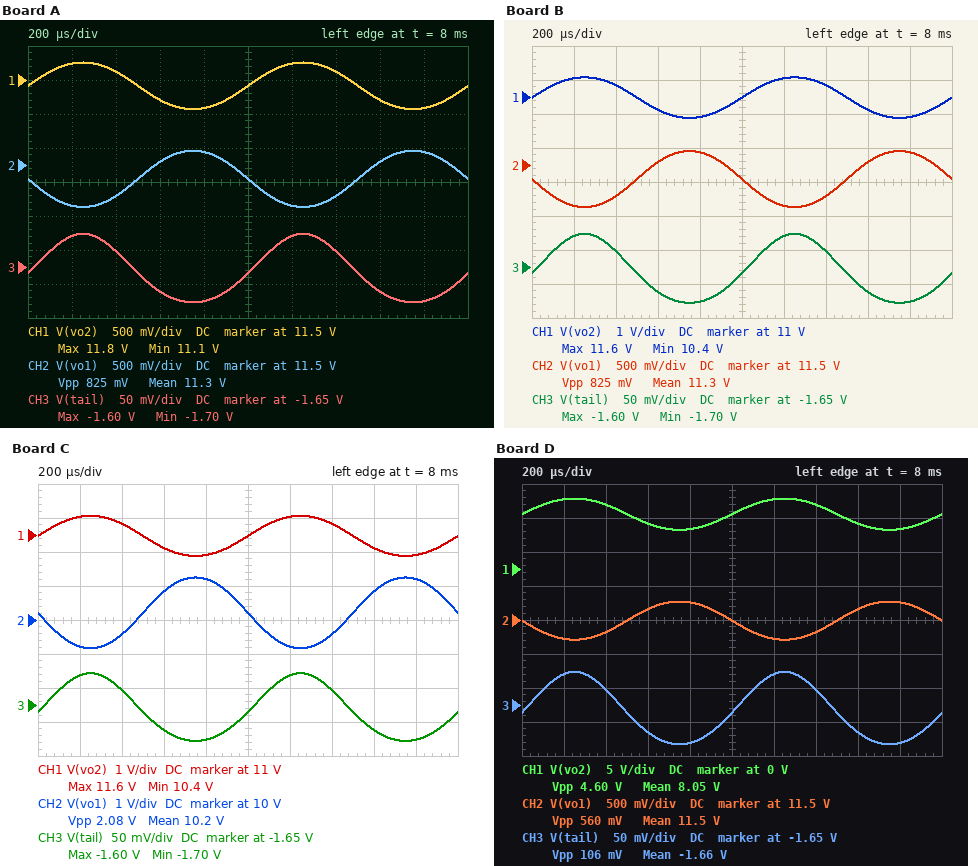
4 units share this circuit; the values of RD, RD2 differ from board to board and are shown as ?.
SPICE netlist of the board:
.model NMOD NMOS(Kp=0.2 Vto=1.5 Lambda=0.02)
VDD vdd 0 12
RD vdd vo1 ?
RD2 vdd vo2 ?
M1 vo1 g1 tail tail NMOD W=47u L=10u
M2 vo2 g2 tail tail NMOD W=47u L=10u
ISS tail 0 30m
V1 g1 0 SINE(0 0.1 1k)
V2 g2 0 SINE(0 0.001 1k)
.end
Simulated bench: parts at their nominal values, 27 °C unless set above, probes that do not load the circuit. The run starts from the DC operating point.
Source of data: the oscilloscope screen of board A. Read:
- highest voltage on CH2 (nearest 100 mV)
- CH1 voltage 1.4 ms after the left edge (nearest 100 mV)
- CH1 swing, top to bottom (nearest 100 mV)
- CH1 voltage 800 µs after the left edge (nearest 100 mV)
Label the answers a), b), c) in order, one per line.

a) 11.7 V
b) 11.6 V
c) 700 mV
d) 11.1 V
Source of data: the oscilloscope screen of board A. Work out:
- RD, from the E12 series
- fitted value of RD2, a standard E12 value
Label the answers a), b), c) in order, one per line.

a) 47 Ω
b) 39 Ω
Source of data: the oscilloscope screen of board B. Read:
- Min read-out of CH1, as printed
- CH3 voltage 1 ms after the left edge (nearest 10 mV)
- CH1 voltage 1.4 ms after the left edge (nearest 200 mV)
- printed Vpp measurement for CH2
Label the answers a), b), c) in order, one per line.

a) 10.4 V
b) -1.66 V
c) 11.4 V
d) 825 mV
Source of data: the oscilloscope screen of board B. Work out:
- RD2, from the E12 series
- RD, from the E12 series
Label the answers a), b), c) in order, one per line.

a) 68 Ω
b) 47 Ω
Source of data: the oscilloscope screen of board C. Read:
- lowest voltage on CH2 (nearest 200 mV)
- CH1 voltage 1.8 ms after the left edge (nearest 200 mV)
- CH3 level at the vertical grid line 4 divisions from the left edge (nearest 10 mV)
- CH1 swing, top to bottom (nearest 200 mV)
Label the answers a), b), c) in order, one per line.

a) 9.2 V
b) 10.4 V
c) -1.70 V
d) 1.2 V
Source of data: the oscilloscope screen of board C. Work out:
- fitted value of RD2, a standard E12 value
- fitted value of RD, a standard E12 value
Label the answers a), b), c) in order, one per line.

a) 68 Ω
b) 120 Ω
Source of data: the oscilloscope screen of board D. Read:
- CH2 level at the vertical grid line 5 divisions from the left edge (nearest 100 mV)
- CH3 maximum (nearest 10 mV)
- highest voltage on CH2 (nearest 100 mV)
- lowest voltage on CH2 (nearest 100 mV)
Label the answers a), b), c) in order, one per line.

a) 11.5 V
b) -1.60 V
c) 11.8 V
d) 11.2 V
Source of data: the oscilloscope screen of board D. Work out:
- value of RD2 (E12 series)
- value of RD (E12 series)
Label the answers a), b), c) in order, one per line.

a) 270 Ω
b) 33 Ω
